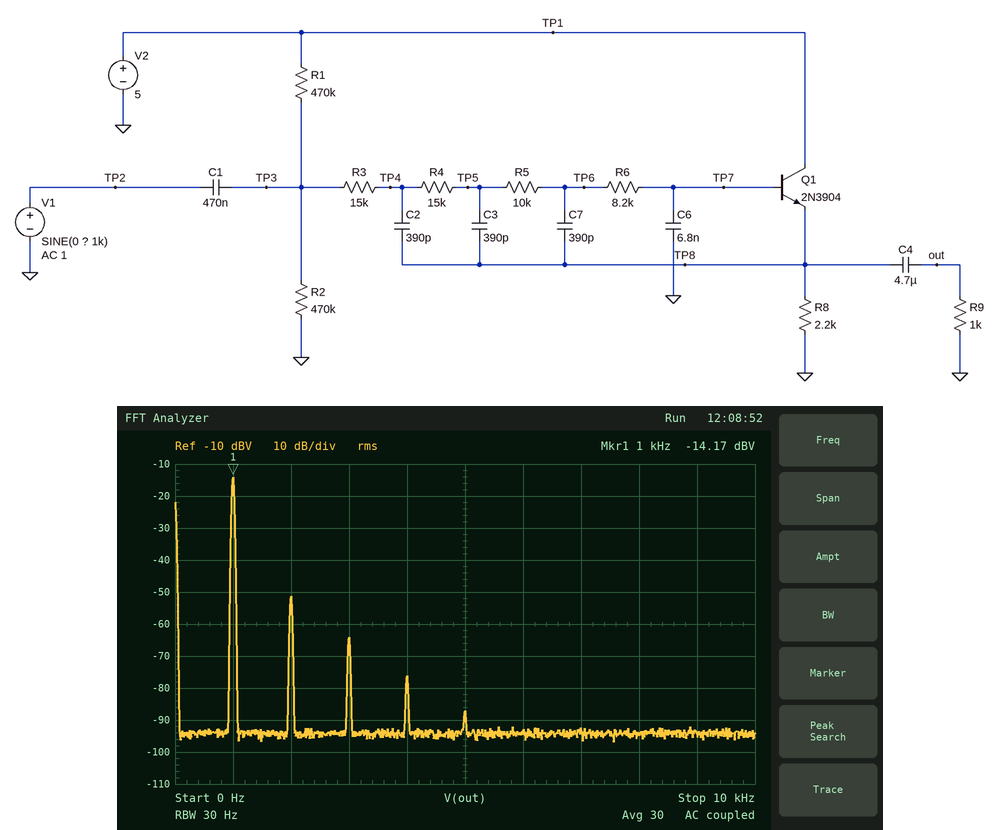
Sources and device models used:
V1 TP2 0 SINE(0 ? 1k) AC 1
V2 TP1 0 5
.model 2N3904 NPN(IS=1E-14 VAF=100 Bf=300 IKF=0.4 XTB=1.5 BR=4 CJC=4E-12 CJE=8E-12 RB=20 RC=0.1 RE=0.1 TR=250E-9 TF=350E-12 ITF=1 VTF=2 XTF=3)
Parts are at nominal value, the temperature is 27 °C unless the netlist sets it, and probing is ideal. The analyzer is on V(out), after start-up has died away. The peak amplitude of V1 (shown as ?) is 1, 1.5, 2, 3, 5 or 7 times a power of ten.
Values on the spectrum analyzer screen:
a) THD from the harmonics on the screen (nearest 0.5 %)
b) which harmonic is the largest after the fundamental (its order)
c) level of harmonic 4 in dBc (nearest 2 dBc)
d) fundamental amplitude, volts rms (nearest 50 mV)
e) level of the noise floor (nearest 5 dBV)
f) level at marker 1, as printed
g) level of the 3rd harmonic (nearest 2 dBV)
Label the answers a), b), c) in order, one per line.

a) 1.5 %
b) 2
c) -62 dBc
d) 200 mV
e) -95 dBV
f) -14.17 dBV
g) -64 dBV
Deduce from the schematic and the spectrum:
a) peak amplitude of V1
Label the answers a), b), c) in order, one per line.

a) 700 mV
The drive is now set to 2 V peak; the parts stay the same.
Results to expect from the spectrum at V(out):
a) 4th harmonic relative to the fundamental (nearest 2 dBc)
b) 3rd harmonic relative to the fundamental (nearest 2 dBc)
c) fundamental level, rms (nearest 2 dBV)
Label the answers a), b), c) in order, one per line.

a) -46 dBc
b) -22 dBc
c) -8 dBV
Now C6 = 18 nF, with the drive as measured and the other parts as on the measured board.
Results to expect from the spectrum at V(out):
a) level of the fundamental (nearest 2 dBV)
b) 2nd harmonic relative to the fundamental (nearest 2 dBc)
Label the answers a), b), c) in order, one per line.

a) -22 dBV
b) -46 dBc
